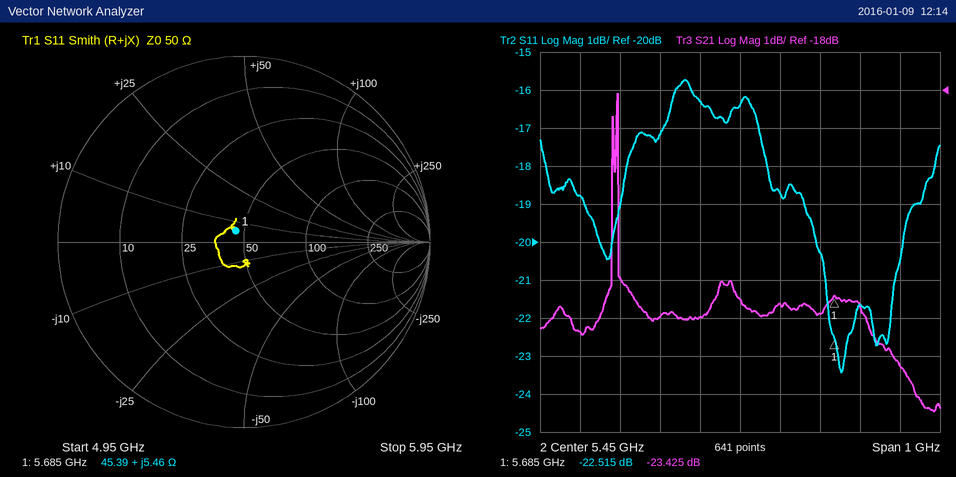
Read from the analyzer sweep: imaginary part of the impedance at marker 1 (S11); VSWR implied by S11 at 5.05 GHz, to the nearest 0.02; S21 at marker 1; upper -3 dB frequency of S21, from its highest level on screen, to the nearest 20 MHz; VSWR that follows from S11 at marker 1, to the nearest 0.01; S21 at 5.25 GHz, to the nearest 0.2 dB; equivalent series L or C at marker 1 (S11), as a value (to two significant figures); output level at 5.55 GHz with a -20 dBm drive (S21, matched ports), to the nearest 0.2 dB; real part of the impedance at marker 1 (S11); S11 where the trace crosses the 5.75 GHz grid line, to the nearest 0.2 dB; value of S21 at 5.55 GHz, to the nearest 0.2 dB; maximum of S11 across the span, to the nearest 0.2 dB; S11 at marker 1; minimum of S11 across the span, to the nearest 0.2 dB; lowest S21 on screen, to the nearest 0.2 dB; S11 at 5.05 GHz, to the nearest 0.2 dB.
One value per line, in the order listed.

+5.46 Ω
1.26
-23.425 dB
5.14 GHz
1.16
-24.0 dB
150 pH
-43.6 dBm
45.39 Ω
-21.6 dB
-23.6 dB
-15.8 dB
-22.515 dB
-23.4 dB
-26.4 dB
-18.8 dB
